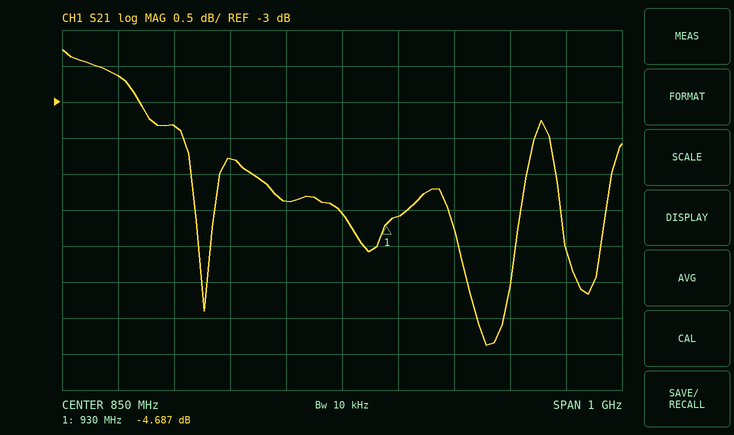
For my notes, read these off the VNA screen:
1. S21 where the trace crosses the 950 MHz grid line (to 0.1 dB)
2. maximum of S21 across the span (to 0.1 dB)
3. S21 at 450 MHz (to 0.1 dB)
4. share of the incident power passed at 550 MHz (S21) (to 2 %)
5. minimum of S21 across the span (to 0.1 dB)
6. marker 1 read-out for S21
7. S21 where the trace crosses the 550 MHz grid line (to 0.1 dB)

-4.6 dB
-2.3 dB
-2.6 dB
46 %
-6.4 dB
-4.687 dB
-3.3 dB
